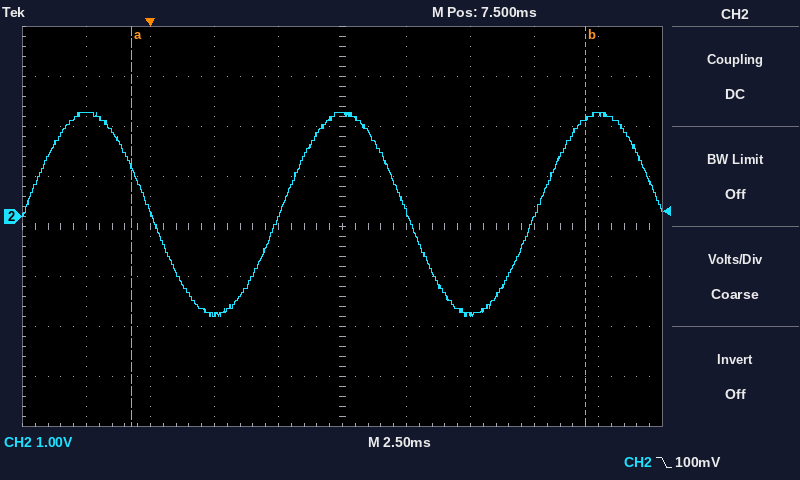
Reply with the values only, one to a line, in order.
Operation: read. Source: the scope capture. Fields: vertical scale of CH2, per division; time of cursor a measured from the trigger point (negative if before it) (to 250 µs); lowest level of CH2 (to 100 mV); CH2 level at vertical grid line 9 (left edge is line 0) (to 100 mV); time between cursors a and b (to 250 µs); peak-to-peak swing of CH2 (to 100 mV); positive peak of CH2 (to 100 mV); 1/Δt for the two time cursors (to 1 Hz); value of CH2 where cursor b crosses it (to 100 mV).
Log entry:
1 V
-750 µs
-2.0 V
2.0 V
17.75 ms
4.1 V
2.1 V
56 Hz
2.0 V
